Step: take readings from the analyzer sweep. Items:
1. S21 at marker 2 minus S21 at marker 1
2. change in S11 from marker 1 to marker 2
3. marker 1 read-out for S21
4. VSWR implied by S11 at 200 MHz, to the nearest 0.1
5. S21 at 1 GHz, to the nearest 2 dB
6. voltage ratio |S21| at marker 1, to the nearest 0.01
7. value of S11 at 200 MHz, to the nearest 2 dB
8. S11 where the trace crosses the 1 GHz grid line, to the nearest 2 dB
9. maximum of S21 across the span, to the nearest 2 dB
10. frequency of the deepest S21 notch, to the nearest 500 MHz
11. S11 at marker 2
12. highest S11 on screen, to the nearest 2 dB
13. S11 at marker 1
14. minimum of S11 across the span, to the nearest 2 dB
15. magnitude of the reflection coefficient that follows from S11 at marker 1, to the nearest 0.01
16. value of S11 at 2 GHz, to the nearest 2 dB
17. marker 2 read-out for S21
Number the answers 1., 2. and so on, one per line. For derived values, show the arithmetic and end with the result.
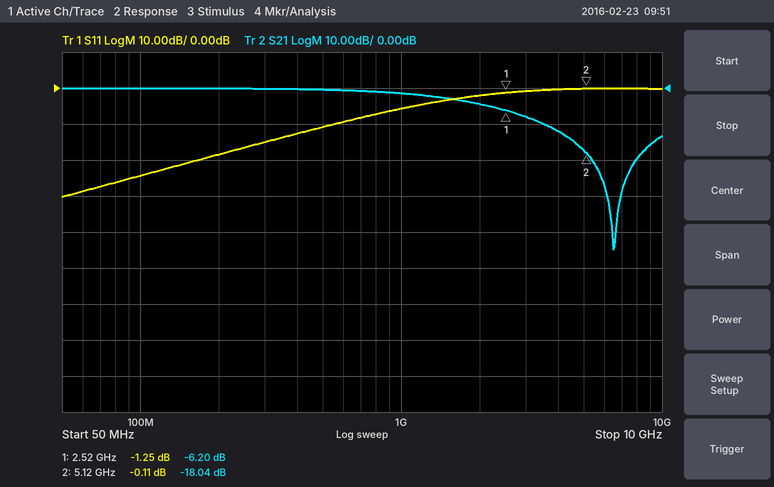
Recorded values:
1. -18.04 − (-6.2) = -11.84 dB
2. -0.11 − (-1.25) = 1.14 dB
3. -6.20 dB
4. |Γ| = 10^(-18/20) = 0.1259; VSWR = (1 + 0.1259)/(1 − 0.1259) ≈ 1.3
5. -2 dB
6. 10^(-6.2/20) ≈ 0.49
7. -18 dB
8. -6 dB
9. 0 dB
10. 6.5 GHz
11. -0.11 dB
12. 0 dB
13. -1.25 dB
14. -30 dB
15. 10^(-1.25/20) ≈ 0.87
16. -2 dB
17. -18.04 dB
